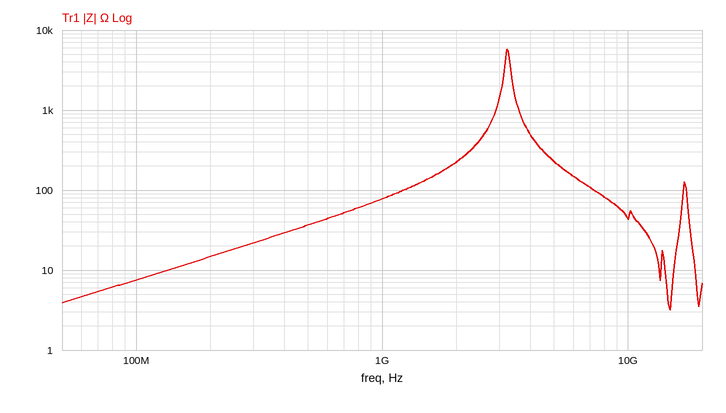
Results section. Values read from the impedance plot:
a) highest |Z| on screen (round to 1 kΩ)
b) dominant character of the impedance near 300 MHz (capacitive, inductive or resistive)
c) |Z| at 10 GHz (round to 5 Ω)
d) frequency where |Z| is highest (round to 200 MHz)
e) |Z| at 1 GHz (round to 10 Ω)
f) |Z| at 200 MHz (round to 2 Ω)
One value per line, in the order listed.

6 kΩ
inductive
45 Ω
3.2 GHz
80 Ω
14 Ω
